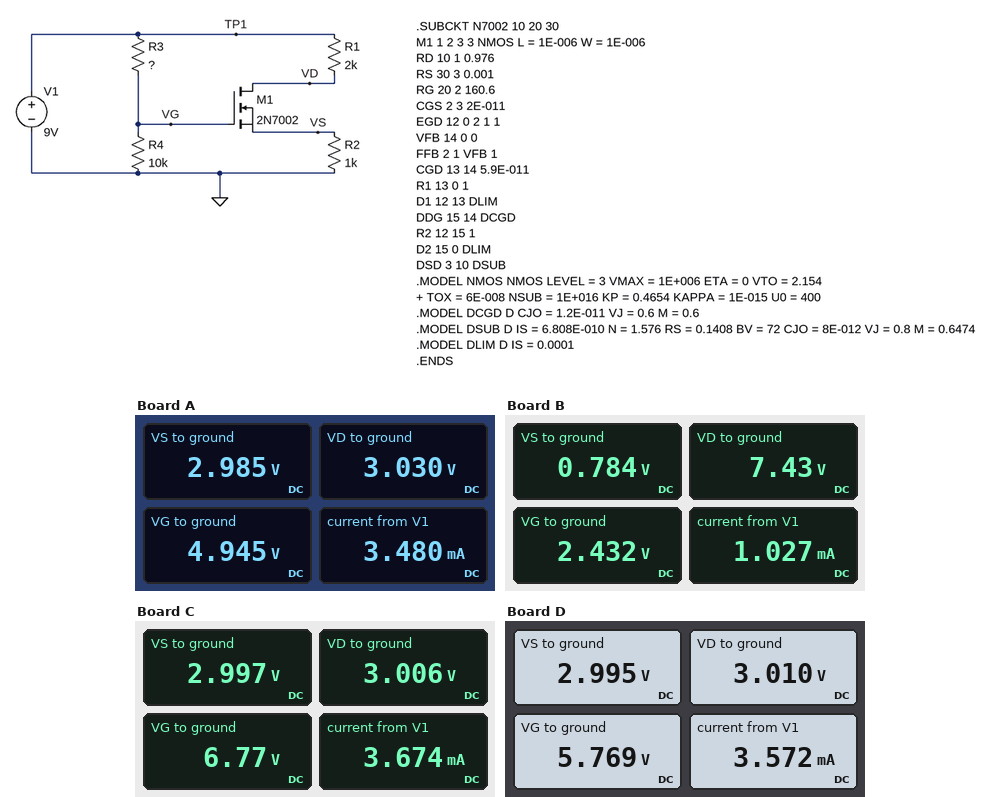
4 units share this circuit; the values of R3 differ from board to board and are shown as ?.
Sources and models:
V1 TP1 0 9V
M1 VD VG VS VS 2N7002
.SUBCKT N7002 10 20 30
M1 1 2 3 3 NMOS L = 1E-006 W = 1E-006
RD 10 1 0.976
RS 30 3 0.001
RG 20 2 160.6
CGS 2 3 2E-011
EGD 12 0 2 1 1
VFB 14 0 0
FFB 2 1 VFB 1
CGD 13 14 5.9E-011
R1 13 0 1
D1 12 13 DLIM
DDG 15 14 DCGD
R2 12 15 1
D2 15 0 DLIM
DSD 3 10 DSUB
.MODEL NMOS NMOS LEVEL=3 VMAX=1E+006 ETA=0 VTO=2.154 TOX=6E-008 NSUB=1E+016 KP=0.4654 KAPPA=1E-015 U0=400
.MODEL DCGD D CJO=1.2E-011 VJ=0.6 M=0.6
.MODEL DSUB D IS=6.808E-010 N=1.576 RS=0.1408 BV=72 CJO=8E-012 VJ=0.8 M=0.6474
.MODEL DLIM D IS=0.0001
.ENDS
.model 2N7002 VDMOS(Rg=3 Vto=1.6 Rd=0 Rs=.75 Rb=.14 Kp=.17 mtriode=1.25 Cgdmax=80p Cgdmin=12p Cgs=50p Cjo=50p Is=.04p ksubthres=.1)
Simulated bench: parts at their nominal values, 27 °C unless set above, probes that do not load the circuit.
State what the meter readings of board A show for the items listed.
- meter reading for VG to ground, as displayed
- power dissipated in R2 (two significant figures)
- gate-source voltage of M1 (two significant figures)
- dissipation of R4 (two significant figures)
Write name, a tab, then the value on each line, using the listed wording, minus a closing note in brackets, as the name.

meter reading for VG to ground, as displayed	4.945 V
power dissipated in R2	8.9 mW
gate-source voltage of M1	2.0 V
dissipation of R4	2.4 mW
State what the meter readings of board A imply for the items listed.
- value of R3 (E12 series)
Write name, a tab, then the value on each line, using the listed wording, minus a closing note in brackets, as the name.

value of R3	8.2 kΩ
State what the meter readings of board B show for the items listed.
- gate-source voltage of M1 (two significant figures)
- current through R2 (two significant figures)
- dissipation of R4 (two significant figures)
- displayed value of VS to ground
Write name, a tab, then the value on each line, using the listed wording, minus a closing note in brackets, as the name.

gate-source voltage of M1	1.6 V
current through R2	780 µA
dissipation of R4	590 µW
displayed value of VS to ground	0.784 V
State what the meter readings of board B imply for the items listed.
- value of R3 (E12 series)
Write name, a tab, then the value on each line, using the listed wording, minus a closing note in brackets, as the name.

value of R3	27 kΩ
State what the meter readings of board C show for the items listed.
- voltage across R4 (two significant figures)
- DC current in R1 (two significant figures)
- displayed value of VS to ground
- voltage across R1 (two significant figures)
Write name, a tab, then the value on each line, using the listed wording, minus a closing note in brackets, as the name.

voltage across R4	6.8 V
DC current in R1	3.0 mA
displayed value of VS to ground	2.997 V
voltage across R1	6.0 V
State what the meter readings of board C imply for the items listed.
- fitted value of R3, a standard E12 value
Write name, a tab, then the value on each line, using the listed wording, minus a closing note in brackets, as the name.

fitted value of R3, a standard E12 value	3.3 kΩ
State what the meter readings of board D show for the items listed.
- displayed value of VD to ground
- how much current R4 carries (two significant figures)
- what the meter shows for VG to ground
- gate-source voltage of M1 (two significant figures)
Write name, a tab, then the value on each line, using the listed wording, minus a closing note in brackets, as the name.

displayed value of VD to ground	3.010 V
how much current R4 carries	580 µA
what the meter shows for VG to ground	5.769 V
gate-source voltage of M1	2.8 V
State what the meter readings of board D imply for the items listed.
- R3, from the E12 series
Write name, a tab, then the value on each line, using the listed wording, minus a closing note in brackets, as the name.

R3, from the E12 series	5.6 kΩ
